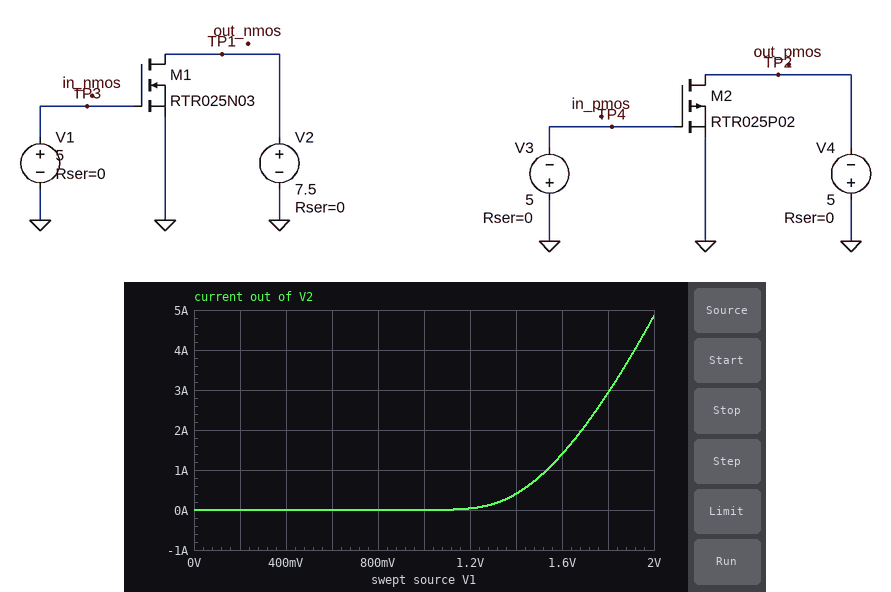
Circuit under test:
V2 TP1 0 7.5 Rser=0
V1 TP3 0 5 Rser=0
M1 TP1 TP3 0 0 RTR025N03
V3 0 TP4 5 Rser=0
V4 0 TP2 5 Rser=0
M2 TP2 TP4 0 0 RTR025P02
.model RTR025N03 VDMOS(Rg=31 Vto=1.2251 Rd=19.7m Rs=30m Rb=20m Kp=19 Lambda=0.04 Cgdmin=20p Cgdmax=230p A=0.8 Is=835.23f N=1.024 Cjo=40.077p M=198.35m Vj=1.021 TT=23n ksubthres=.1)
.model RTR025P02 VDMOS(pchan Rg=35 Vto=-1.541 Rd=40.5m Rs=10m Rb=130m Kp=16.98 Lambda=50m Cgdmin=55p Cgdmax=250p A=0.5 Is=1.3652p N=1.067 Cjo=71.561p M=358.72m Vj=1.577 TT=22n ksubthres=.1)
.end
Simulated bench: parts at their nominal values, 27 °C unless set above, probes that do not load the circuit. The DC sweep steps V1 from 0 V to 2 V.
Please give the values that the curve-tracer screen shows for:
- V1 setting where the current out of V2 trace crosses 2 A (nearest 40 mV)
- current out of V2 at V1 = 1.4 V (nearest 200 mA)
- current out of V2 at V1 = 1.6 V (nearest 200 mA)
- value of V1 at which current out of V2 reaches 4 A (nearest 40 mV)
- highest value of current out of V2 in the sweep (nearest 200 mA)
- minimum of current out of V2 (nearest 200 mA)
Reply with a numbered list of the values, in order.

1. 1.68 V
2. 400 mA
3. 1.4 A
4. 1.92 V
5. 4.8 A
6. 0 A
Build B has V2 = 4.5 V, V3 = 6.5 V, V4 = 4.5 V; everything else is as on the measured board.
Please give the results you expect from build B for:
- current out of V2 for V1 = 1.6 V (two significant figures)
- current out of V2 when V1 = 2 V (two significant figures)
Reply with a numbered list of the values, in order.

1. 1.3 A
2. 4.5 A
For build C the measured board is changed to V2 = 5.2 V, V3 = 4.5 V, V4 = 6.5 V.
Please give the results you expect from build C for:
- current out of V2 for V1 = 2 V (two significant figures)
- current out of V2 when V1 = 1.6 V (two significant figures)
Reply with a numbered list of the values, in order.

1. 4.6 A
2. 1.3 A
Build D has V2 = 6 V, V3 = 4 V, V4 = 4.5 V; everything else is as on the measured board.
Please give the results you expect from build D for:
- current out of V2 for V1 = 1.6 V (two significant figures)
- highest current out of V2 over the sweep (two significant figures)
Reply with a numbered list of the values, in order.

1. 1.3 A
2. 4.7 A
